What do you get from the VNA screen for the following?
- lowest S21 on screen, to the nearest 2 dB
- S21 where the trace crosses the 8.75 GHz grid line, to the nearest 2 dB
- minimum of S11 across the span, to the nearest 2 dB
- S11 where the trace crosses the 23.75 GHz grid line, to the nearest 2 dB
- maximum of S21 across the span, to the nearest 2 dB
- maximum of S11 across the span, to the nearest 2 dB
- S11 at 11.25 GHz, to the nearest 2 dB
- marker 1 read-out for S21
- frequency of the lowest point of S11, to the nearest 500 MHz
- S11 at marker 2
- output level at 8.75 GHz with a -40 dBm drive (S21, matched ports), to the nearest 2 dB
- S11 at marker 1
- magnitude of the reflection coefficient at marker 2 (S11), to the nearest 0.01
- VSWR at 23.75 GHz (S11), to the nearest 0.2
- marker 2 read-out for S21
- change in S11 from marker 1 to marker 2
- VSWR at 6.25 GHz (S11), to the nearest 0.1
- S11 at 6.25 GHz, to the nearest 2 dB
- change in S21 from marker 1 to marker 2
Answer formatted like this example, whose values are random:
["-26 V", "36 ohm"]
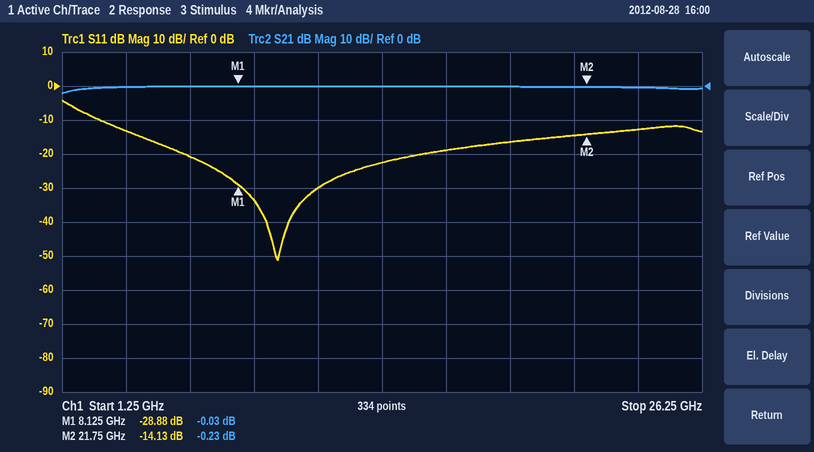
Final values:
["-2 dB", "0 dB", "-52 dB", "-12 dB", "0 dB", "-4 dB", "-30 dB", "-0.03 dB", "9.5 GHz", "-14.13 dB", "-40 dBm", "-28.88 dB", "0.20", "1.6", "-0.23 dB", "14.75 dB", "1.2", "-20 dB", "-0.20 dB"]
